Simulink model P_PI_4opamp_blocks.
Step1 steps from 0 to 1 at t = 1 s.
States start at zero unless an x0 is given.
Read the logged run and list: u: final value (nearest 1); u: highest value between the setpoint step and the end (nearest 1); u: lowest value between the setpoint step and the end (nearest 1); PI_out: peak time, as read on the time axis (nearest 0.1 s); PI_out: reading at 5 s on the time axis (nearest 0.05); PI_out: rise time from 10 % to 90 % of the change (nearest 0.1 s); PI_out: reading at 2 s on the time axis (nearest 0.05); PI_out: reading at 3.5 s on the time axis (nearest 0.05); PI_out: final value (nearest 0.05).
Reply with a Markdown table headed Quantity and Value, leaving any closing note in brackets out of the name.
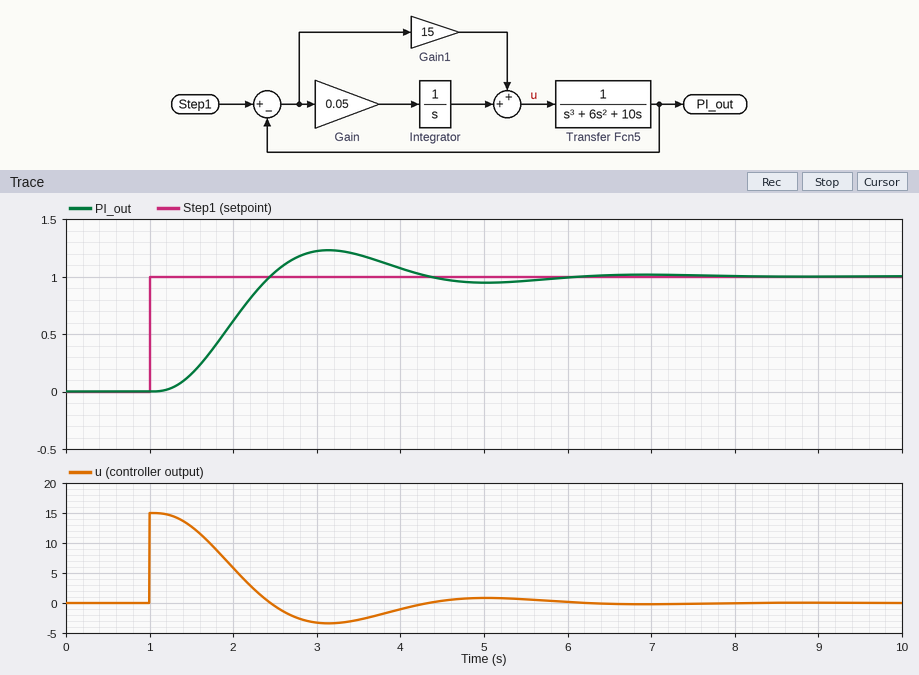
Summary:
| Quantity | Value |
|---|---|
| u: final value | 0 |
| u: highest value between the setpoint step and the end | 15 |
| u: lowest value between the setpoint step and the end | -3 |
| PI_out: peak time, as read on the time axis | 3.1 s |
| PI_out: reading at 5 s on the time axis | 0.95 |
| PI_out: rise time from 10 % to 90 % of the change | 0.9 s |
| PI_out: reading at 2 s on the time axis | 0.60 |
| PI_out: reading at 3.5 s on the time axis | 1.20 |
| PI_out: final value | 1.00 |
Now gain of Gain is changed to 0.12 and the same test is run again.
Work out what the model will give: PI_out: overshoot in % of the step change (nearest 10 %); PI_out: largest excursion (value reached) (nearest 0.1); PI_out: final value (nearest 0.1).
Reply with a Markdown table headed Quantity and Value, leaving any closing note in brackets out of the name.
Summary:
| Quantity | Value |
|---|---|
| PI_out: overshoot in % of the step change | 20 % |
| PI_out: largest excursion (value reached) | 1.2 |
| PI_out: final value | 1.0 |
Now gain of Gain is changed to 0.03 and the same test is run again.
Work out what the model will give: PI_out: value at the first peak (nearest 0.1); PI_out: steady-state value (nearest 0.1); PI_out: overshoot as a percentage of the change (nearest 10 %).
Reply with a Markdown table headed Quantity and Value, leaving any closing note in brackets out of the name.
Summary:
| Quantity | Value |
|---|---|
| PI_out: value at the first peak | 1.2 |
| PI_out: steady-state value | 1.0 |
| PI_out: overshoot as a percentage of the change | 20 % |
